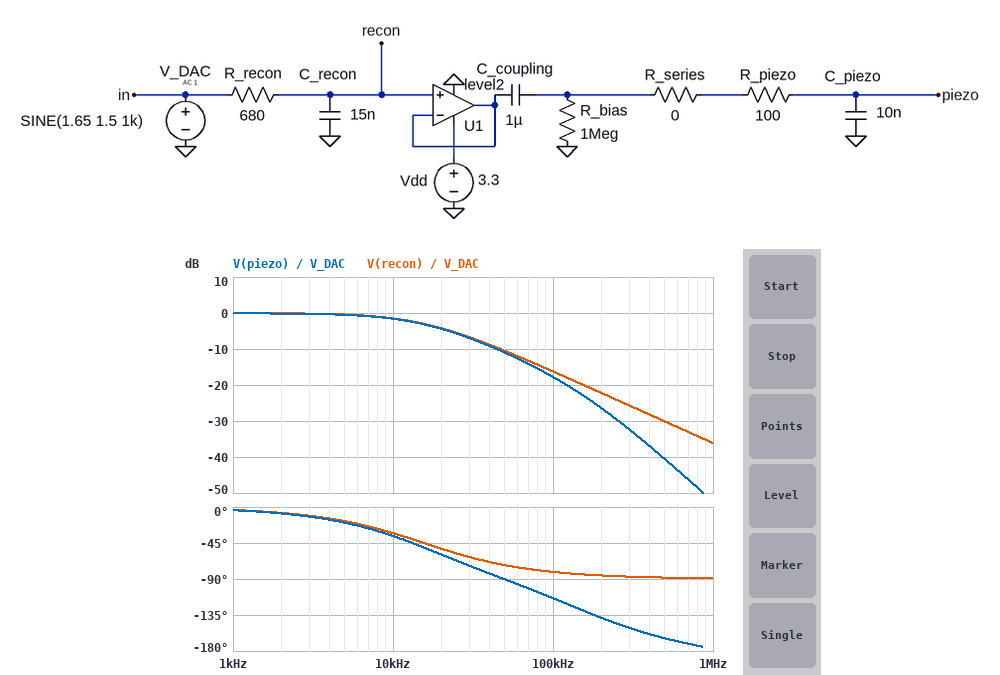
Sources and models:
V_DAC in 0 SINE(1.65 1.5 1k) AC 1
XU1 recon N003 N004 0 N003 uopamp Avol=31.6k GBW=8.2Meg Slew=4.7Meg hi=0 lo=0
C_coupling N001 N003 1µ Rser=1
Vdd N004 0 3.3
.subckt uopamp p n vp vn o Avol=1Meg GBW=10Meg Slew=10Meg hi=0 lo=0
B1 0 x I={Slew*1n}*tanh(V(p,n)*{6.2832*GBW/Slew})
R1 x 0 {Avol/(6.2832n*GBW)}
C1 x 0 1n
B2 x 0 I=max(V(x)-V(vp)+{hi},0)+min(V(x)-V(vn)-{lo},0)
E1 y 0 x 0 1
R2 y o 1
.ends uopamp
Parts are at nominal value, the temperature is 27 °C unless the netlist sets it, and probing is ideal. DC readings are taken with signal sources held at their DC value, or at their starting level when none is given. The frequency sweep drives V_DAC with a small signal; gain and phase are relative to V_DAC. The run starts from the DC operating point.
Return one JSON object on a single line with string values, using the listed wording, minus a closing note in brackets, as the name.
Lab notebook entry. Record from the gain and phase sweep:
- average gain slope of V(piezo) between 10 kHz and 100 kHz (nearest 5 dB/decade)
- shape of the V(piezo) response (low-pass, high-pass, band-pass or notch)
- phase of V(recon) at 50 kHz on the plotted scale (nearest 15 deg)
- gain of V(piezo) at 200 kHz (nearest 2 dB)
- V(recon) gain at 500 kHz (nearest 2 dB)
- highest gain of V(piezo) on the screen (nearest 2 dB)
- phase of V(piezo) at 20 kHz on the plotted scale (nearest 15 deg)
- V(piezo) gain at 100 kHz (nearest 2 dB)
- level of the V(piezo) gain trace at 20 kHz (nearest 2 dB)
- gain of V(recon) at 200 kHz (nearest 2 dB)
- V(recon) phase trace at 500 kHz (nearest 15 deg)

{"average gain slope of V(piezo) between 10 kHz and 100 kHz": "-15 dB/decade", "shape of the V(piezo) response": "low-pass", "phase of V(recon) at 50 kHz on the plotted scale": "-75 deg", "gain of V(piezo) at 200 kHz": "-26 dB", "V(recon) gain at 500 kHz": "-30 dB", "highest gain of V(piezo) on the screen": "0 dB", "phase of V(piezo) at 20 kHz on the plotted scale": "-60 deg", "V(piezo) gain at 100 kHz": "-18 dB", "level of the V(piezo) gain trace at 20 kHz": "-4 dB", "gain of V(recon) at 200 kHz": "-22 dB", "V(recon) phase trace at 500 kHz": "-90 deg"}
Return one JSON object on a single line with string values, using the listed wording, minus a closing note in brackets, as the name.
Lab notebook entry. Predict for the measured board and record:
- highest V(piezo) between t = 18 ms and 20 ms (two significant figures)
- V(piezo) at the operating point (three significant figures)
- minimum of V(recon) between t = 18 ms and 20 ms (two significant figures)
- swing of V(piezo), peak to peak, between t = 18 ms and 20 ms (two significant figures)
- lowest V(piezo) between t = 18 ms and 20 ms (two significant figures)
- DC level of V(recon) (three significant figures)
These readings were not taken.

{"highest V(piezo) between t = 18 ms and 20 ms": "1.5 V", "V(piezo) at the operating point": "1.63 V", "minimum of V(recon) between t = 18 ms and 20 ms": "150 mV", "swing of V(piezo), peak to peak, between t = 18 ms and 20 ms": "3.0 V", "lowest V(piezo) between t = 18 ms and 20 ms": "-1.5 V", "DC level of V(recon)": "1.65 V"}
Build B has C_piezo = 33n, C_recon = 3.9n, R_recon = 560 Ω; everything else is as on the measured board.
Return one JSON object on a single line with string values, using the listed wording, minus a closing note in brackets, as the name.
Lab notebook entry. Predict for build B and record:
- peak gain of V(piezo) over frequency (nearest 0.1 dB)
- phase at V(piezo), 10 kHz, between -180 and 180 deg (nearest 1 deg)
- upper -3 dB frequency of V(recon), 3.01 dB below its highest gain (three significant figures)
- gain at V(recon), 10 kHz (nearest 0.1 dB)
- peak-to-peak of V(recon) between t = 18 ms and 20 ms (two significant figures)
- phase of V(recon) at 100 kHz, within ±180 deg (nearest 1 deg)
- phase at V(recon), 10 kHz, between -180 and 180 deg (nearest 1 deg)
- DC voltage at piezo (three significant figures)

{"peak gain of V(piezo) over frequency": "-0.3 dB", "phase at V(piezo), 10 kHz, between -180 and 180 deg": "-19 deg", "upper -3 dB frequency of V(recon), 3.01 dB below its highest gain": "72.9 kHz", "gain at V(recon), 10 kHz": "-0.1 dB", "peak-to-peak of V(recon) between t = 18 ms and 20 ms": "3.0 V", "phase of V(recon) at 100 kHz, within ±180 deg": "-54 deg", "phase at V(recon), 10 kHz, between -180 and 180 deg": "-8 deg", "DC voltage at piezo": "1.52 V"}
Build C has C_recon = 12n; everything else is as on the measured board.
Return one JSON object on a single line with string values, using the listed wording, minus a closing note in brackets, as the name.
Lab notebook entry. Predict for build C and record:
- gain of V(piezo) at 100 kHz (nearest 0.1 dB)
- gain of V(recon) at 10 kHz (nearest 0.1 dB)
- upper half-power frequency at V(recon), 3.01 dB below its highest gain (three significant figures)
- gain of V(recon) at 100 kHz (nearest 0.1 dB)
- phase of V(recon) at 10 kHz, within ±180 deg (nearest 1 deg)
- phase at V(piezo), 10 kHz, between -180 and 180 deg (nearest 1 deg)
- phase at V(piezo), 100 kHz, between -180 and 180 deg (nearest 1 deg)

{"gain of V(piezo) at 100 kHz": "-15.9 dB", "gain of V(recon) at 10 kHz": "-1.0 dB", "upper half-power frequency at V(recon), 3.01 dB below its highest gain": "19.5 kHz", "gain of V(recon) at 100 kHz": "-14.4 dB", "phase of V(recon) at 10 kHz, within ±180 deg": "-27 deg", "phase at V(piezo), 10 kHz, between -180 and 180 deg": "-31 deg", "phase at V(piezo), 100 kHz, between -180 and 180 deg": "-112 deg"}
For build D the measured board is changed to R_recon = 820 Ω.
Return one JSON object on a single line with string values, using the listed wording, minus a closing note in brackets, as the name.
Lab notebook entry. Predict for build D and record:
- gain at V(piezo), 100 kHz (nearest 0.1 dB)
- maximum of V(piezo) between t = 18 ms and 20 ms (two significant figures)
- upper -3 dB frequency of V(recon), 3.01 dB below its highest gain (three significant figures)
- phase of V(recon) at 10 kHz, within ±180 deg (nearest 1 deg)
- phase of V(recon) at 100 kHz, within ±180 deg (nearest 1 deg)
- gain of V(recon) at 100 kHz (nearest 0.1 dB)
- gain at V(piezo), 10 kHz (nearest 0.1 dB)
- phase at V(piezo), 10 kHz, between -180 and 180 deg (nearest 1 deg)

{"gain at V(piezo), 100 kHz": "-19.4 dB", "maximum of V(piezo) between t = 18 ms and 20 ms": "1.5 V", "upper -3 dB frequency of V(recon), 3.01 dB below its highest gain": "12.9 kHz", "phase of V(recon) at 10 kHz, within ±180 deg": "-38 deg", "phase of V(recon) at 100 kHz, within ±180 deg": "-83 deg", "gain of V(recon) at 100 kHz": "-17.8 dB", "gain at V(piezo), 10 kHz": "-2.1 dB", "phase at V(piezo), 10 kHz, between -180 and 180 deg": "-41 deg"}
